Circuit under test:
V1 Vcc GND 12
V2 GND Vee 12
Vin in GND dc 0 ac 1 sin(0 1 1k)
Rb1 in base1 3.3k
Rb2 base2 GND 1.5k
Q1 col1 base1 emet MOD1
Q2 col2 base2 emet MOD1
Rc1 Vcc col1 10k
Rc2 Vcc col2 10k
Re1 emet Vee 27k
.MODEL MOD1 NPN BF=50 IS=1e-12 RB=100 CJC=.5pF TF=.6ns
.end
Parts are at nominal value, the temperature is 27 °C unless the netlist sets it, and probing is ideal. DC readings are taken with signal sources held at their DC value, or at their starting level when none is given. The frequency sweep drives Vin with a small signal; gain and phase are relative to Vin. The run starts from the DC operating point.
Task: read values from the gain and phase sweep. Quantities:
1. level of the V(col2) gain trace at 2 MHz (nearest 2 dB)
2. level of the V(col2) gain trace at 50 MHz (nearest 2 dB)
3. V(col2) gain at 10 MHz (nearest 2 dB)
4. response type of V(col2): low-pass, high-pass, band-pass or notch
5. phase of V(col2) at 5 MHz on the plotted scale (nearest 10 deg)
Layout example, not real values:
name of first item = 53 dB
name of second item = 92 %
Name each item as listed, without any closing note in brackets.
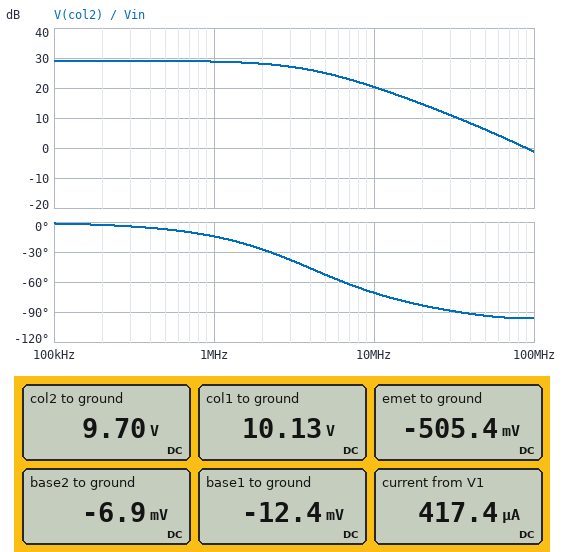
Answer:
level of the V(col2) gain trace at 2 MHz = 28 dB
level of the V(col2) gain trace at 50 MHz = 6 dB
V(col2) gain at 10 MHz = 20 dB
response type of V(col2): low-pass, high-pass, band-pass or notch = low-pass
phase of V(col2) at 5 MHz on the plotted scale = -50 deg
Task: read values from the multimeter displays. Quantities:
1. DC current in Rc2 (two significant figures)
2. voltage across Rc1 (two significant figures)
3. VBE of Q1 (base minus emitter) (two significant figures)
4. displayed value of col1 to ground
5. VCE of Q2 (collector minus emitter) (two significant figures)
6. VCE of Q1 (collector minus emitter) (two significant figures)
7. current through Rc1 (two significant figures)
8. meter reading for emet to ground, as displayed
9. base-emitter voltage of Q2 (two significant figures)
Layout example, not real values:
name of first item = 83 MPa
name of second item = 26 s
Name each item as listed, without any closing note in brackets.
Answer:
DC current in Rc2 = 230 µA
voltage across Rc1 = 1.9 V
VBE of Q1 (base minus emitter) = 490 mV
displayed value of col1 to ground = 10.13 V
VCE of Q2 (collector minus emitter) = 10 V
VCE of Q1 (collector minus emitter) = 11 V
current through Rc1 = 190 µA
meter reading for emet to ground, as displayed = -505.4 mV
base-emitter voltage of Q2 = 500 mV
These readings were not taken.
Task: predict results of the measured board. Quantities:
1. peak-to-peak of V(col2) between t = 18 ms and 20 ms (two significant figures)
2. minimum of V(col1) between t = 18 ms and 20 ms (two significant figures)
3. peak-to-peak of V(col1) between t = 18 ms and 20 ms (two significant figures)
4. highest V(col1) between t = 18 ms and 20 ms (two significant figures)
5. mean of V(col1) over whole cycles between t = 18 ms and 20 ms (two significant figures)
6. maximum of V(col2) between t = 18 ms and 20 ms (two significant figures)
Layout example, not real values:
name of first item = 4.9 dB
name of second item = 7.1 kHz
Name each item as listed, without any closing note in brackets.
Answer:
peak-to-peak of V(col2) between t = 18 ms and 20 ms = 4.2 V
minimum of V(col1) between t = 18 ms and 20 ms = 7.5 V
peak-to-peak of V(col1) between t = 18 ms and 20 ms = 4.5 V
highest V(col1) between t = 18 ms and 20 ms = 12 V
mean of V(col1) over whole cycles between t = 18 ms and 20 ms = 9.8 V
maximum of V(col2) between t = 18 ms and 20 ms = 12 V
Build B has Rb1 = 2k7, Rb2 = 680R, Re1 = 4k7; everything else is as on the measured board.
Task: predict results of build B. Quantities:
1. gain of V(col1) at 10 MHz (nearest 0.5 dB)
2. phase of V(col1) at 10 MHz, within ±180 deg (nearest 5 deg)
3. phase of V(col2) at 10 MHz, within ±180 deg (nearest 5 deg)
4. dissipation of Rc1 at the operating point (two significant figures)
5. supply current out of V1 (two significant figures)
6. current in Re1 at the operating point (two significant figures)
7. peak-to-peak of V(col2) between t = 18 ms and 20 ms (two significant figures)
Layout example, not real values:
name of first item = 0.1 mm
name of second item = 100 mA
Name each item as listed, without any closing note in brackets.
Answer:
gain of V(col1) at 10 MHz = 18.5 dB
phase of V(col1) at 10 MHz, within ±180 deg = 125 deg
phase of V(col2) at 10 MHz, within ±180 deg = -40 deg
dissipation of Rc1 at the operating point = 12 mW
supply current out of V1 = 2.3 mA
current in Re1 at the operating point = 2.4 mA
peak-to-peak of V(col2) between t = 18 ms and 20 ms = 5.1 V
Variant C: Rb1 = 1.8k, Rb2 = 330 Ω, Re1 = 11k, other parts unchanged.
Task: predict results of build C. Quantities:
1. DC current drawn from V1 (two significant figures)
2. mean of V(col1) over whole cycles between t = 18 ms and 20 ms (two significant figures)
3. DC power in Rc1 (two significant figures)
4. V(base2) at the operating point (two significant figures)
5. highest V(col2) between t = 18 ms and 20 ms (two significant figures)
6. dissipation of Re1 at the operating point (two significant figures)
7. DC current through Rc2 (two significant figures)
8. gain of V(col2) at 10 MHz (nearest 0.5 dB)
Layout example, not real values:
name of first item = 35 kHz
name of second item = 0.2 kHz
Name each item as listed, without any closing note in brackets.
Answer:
DC current drawn from V1 = 1.0 mA
mean of V(col1) over whole cycles between t = 18 ms and 20 ms = 6.7 V
DC power in Rc1 = 1.7 mW
V(base2) at the operating point = -4.0 mV
highest V(col2) between t = 18 ms and 20 ms = 12 V
dissipation of Re1 at the operating point = 12 mW
DC current through Rc2 = 610 µA
gain of V(col2) at 10 MHz = 26.5 dB
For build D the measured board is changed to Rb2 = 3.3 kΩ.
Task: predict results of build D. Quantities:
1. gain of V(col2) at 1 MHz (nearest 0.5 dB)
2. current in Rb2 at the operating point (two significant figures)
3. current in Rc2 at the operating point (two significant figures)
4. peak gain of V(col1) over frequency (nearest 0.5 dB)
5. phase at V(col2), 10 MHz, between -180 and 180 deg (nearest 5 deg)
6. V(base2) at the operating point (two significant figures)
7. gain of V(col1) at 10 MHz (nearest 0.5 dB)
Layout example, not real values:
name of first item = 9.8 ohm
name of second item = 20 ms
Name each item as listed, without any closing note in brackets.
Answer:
gain of V(col2) at 1 MHz = 28.0 dB
current in Rb2 at the operating point = 4.2 µA
current in Rc2 at the operating point = 210 µA
peak gain of V(col1) over frequency = 28.5 dB
phase at V(col2), 10 MHz, between -180 and 180 deg = -75 deg
V(base2) at the operating point = -14 mV
gain of V(col1) at 10 MHz = 18.0 dB
